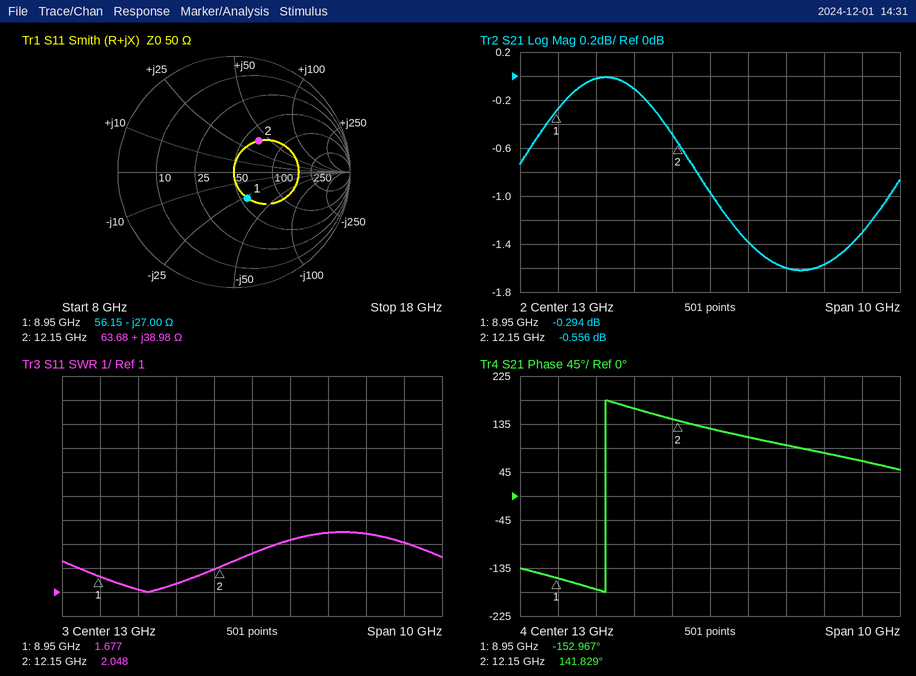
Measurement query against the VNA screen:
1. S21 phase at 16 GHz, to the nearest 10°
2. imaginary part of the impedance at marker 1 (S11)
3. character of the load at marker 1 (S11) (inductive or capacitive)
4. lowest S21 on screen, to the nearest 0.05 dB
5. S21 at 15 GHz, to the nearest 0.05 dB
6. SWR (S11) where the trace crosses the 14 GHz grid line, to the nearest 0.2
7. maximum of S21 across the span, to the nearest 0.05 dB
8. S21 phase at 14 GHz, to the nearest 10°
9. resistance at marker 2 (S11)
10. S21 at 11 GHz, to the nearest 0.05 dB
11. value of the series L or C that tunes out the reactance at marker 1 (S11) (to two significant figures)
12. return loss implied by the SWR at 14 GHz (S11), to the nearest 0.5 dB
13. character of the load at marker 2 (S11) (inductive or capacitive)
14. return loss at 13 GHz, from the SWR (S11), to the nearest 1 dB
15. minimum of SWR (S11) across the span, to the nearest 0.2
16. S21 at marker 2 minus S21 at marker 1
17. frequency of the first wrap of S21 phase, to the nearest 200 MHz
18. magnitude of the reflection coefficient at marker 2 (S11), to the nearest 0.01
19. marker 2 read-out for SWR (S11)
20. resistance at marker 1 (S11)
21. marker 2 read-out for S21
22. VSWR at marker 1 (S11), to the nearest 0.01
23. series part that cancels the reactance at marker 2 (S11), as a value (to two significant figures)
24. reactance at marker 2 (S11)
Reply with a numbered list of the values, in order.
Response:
1. 80°
2. -27.00 Ω
3. capacitive
4. -1.60 dB
5. -1.60 dB
6. 3.2
7. 0.00 dB
8. 110°
9. 63.68 Ω
10. -0.10 dB
11. 480 pH
12. 5.5 dB
13. inductive
14. 7 dB
15. 1.0
16. -0.262 dB
17. 10.2 GHz
18. 0.34
19. 2.048
20. 56.15 Ω
21. -0.556 dB
22. 1.68
23. 340 fF
24. +38.98 Ω
